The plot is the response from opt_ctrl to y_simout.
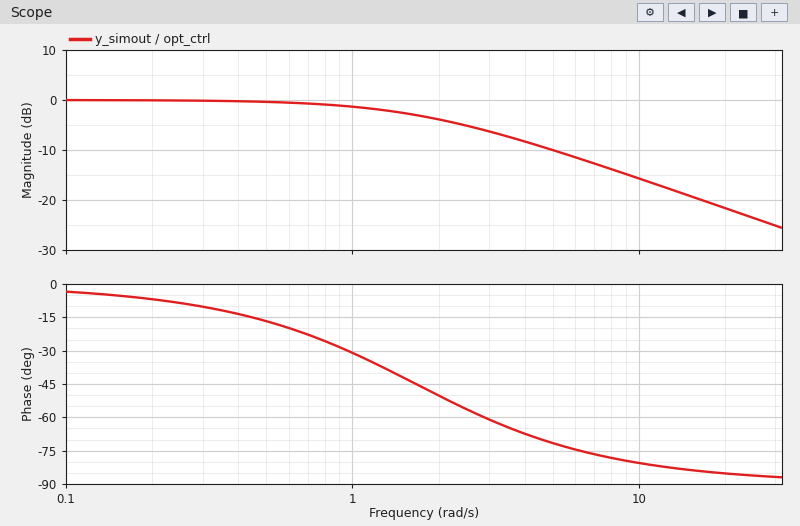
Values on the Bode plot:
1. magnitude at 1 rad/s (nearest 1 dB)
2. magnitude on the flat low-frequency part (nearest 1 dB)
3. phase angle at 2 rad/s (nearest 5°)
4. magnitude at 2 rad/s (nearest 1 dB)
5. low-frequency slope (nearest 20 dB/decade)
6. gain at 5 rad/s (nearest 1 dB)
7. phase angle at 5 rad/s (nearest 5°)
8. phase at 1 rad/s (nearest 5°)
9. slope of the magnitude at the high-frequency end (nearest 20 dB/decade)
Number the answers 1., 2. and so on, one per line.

1. -1 dB
2. 0 dB
3. -50°
4. -4 dB
5. 0 dB/decade
6. -10 dB
7. -70°
8. -30°
9. -20 dB/decade
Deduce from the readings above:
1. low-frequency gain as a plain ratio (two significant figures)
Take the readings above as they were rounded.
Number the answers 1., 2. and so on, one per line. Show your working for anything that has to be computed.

1. 10^(0 / 20) = 1.0
